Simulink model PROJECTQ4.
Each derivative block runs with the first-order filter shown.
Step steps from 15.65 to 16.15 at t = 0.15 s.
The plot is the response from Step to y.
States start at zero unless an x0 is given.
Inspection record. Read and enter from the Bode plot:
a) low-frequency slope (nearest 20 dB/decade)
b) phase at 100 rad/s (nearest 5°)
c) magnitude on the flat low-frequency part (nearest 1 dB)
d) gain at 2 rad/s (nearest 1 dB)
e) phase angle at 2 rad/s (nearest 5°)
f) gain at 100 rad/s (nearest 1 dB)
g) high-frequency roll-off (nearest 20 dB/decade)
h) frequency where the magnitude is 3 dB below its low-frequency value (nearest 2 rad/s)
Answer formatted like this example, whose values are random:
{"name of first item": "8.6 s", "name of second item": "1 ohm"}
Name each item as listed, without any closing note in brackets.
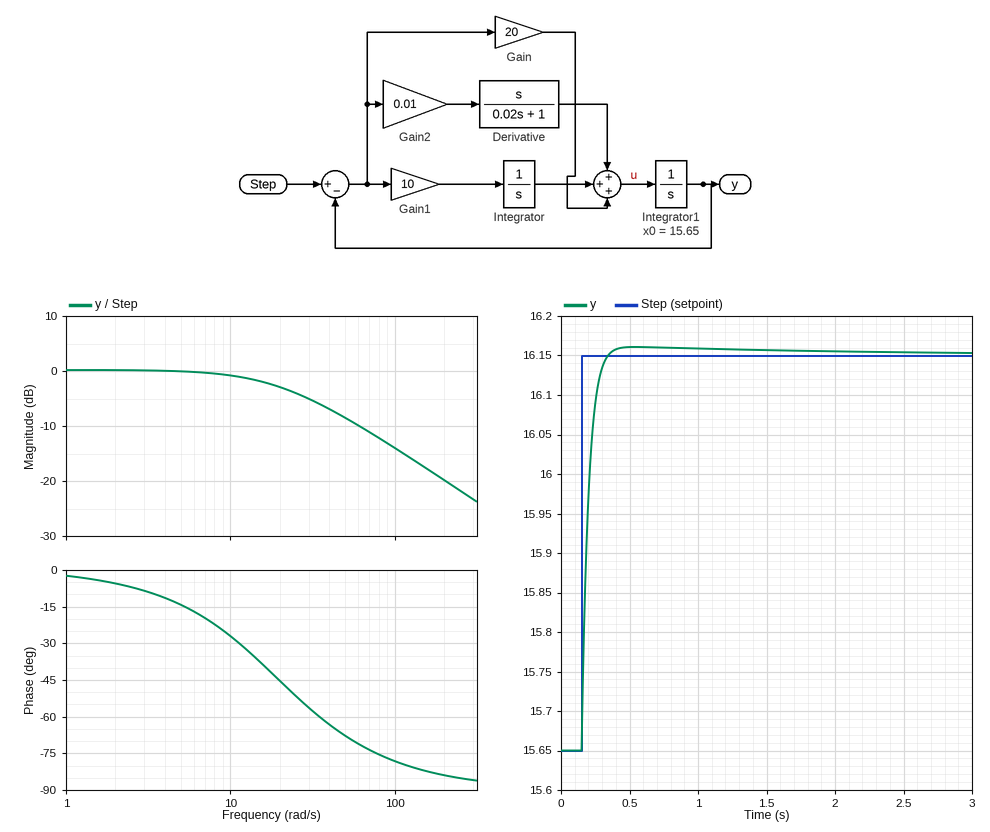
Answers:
{"low-frequency slope": "0 dB/decade", "phase at 100 rad/s": "-80°", "magnitude on the flat low-frequency part": "0 dB", "gain at 2 rad/s": "0 dB", "phase angle at 2 rad/s": "-5°", "gain at 100 rad/s": "-14 dB", "high-frequency roll-off": "-20 dB/decade", "frequency where the magnitude is 3 dB below its low-frequency value": "20 rad/s"}
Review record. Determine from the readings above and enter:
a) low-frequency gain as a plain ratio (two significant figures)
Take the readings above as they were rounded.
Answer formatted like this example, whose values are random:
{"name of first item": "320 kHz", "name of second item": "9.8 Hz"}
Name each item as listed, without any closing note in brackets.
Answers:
{"low-frequency gain as a plain ratio": "1.0"}
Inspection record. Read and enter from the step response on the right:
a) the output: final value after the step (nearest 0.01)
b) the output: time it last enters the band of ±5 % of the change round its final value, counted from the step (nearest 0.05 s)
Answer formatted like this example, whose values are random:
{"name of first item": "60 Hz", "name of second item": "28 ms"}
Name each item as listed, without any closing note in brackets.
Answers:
{"the output: final value after the step": "16.15", "the output: time it last enters the band of ±5 % of the change round its final value, counted from the step": "0.15 s"}
